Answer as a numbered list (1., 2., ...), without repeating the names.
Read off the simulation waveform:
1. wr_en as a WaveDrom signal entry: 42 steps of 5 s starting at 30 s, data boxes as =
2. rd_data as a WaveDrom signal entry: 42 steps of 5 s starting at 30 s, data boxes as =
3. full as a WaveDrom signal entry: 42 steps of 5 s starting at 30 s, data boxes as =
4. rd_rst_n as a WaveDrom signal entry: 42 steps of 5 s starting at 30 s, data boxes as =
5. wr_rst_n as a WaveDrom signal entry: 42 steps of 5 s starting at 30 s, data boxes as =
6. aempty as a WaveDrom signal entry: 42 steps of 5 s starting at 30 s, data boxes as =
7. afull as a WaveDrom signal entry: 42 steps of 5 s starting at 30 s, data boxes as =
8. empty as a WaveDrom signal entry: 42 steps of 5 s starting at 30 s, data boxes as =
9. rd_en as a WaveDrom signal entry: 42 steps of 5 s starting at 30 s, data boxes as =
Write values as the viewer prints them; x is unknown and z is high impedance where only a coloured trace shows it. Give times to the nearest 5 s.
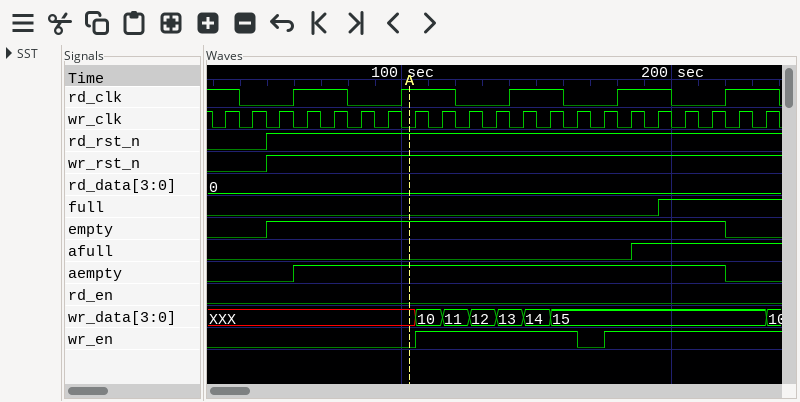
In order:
1. {name: 'wr_en', wave: '0..............1...........0.1............'}
2. {name: 'rd_data', wave: '=.........................................', data: '0'}
3. {name: 'full', wave: '0................................1........'}
4. {name: 'rd_rst_n', wave: '0...1.....................................'}
5. {name: 'wr_rst_n', wave: '0...1.....................................'}
6. {name: 'aempty', wave: '0.....1...............................0...'}
7. {name: 'afull', wave: '0..............................1..........'}
8. {name: 'empty', wave: '0...1.................................0...'}
9. {name: 'rd_en', wave: '0.........................................'}
